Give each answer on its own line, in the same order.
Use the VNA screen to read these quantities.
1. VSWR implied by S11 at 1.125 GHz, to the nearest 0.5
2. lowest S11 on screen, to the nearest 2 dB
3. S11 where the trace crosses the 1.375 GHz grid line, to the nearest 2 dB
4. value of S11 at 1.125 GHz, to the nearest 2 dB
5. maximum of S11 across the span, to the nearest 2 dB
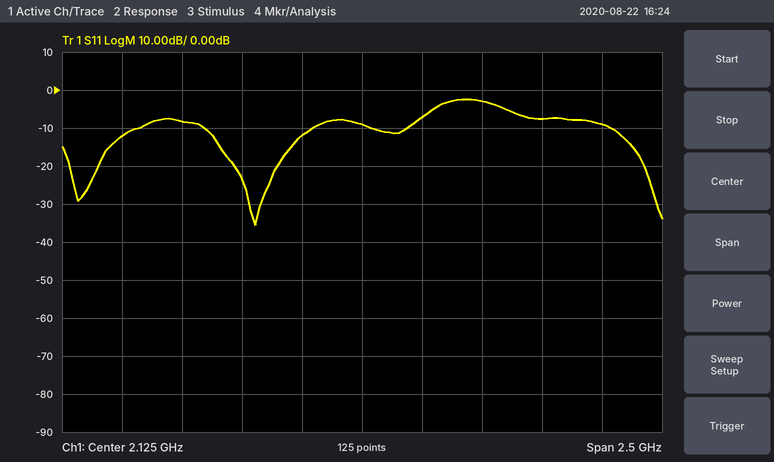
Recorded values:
1.5
-36 dB
-8 dB
-12 dB
-2 dB
